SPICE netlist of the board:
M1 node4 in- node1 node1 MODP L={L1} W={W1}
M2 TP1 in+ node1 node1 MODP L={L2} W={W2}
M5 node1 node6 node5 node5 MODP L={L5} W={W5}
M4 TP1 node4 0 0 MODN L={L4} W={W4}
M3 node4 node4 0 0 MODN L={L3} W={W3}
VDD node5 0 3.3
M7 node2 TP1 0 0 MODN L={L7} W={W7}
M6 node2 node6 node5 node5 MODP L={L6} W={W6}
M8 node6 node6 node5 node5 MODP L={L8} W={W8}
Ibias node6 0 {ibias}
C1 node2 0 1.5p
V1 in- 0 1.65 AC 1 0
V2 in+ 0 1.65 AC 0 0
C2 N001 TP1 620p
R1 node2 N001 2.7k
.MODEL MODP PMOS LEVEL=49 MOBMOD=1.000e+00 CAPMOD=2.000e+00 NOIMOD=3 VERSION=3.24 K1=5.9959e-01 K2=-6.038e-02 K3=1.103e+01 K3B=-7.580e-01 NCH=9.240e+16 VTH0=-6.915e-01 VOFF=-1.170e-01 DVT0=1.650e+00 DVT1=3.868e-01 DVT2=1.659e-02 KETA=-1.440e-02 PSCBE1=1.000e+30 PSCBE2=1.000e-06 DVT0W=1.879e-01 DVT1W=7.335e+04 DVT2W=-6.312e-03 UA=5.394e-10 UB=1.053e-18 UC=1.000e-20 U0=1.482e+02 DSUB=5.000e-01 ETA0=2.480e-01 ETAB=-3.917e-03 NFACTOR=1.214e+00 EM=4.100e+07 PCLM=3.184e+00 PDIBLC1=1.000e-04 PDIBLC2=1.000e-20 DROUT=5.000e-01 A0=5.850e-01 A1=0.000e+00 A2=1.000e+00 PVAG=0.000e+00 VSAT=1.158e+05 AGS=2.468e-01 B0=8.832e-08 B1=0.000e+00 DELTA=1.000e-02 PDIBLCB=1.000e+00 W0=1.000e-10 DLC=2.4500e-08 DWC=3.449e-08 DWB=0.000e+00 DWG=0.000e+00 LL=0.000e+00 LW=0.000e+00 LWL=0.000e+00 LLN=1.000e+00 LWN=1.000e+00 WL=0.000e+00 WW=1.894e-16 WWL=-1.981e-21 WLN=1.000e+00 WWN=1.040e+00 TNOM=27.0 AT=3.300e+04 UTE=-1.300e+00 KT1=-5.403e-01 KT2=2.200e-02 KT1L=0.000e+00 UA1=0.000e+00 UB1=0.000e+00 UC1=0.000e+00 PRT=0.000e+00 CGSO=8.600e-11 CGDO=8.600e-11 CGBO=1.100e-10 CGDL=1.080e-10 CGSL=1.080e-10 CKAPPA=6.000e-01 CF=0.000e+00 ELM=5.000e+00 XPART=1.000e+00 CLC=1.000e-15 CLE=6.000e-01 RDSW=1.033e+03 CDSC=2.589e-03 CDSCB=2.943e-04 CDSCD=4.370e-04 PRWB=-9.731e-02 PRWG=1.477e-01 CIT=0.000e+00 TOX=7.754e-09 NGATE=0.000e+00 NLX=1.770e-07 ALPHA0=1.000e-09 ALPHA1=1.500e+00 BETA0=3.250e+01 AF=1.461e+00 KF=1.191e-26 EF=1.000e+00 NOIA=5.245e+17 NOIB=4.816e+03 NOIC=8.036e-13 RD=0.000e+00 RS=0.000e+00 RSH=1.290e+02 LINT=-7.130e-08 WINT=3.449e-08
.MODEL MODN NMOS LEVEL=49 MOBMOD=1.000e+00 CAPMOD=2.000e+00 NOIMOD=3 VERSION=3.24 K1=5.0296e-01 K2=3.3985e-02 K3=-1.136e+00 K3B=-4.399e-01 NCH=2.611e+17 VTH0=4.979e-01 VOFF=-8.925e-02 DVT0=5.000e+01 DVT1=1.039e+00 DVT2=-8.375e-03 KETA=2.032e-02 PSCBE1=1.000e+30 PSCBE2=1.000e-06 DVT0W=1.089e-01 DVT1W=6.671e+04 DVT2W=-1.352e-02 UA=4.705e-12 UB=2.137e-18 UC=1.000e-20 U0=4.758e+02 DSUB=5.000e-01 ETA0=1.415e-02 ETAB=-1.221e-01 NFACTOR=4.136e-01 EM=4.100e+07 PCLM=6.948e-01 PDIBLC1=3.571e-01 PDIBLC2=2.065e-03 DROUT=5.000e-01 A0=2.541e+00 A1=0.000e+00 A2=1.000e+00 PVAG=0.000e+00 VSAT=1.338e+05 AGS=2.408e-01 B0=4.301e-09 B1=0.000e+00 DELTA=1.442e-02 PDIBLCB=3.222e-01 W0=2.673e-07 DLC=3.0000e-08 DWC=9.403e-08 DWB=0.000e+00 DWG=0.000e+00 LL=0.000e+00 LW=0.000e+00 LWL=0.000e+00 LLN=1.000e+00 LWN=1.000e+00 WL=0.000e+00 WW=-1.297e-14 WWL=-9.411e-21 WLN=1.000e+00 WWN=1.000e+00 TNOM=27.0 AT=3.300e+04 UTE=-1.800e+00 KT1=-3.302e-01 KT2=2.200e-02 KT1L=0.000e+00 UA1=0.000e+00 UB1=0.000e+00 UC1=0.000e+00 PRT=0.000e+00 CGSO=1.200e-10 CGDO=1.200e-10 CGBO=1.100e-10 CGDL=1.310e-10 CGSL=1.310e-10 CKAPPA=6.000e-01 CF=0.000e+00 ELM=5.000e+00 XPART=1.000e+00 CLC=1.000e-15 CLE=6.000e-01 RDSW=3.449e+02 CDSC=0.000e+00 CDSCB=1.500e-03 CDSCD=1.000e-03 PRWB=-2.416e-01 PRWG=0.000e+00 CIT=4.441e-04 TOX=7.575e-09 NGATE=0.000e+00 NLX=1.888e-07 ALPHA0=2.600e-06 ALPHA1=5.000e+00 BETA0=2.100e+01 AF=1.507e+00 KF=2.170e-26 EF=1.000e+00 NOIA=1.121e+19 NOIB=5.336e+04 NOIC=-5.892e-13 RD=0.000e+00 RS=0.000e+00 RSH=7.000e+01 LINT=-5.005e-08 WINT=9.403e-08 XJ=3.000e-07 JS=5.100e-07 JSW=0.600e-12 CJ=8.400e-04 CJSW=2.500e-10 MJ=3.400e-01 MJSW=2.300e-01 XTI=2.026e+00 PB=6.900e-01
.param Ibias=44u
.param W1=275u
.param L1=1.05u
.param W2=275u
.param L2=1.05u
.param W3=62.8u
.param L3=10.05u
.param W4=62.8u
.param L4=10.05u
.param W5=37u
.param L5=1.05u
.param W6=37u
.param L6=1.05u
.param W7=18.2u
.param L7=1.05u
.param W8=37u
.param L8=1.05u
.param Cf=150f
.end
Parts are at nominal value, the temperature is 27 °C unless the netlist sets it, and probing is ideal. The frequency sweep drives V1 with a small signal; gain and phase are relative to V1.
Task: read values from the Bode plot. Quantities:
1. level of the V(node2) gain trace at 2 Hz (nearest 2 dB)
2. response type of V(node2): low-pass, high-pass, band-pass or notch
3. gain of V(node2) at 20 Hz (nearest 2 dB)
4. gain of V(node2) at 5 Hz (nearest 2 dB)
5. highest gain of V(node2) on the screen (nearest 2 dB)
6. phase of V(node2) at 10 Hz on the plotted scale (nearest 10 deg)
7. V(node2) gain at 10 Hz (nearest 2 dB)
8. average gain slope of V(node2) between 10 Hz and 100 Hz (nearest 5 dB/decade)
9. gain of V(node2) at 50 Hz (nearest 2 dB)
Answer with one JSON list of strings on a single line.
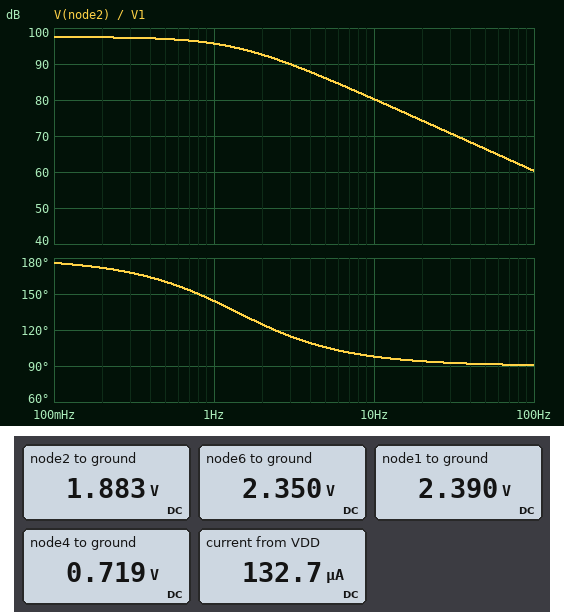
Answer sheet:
["92 dB", "low-pass", "74 dB", "86 dB", "98 dB", "100 deg", "80 dB", "-20 dB/decade", "66 dB"]
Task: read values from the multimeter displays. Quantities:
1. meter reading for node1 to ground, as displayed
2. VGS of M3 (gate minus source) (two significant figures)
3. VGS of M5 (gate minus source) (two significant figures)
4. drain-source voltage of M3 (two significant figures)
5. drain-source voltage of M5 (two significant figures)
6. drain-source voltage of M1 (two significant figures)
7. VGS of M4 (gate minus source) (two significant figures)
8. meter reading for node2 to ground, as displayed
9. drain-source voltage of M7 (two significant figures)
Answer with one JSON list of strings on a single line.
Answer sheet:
["2.390 V", "720 mV", "-950 mV", "720 mV", "-910 mV", "-1.7 V", "720 mV", "1.883 V", "1.9 V"]
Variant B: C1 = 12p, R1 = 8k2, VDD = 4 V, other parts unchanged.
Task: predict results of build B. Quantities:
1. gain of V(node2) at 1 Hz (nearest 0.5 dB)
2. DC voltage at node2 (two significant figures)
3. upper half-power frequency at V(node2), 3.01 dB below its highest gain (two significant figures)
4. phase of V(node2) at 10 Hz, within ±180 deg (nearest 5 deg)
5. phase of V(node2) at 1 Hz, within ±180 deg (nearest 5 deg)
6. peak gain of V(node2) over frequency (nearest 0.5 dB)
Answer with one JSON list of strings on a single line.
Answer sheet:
["97.0 dB", "1.7 V", "1.1 Hz", "95 deg", "140 deg", "99.5 dB"]
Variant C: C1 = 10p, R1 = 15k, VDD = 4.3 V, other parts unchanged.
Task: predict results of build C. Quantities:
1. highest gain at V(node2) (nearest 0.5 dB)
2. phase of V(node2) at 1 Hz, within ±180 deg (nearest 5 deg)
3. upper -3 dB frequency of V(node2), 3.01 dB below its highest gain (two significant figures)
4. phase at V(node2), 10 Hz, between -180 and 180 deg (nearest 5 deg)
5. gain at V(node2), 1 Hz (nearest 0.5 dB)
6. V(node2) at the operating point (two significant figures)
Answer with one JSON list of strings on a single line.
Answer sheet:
["100.0 dB", "135 deg", "1.1 Hz", "95 deg", "97.0 dB", "1.6 V"]
